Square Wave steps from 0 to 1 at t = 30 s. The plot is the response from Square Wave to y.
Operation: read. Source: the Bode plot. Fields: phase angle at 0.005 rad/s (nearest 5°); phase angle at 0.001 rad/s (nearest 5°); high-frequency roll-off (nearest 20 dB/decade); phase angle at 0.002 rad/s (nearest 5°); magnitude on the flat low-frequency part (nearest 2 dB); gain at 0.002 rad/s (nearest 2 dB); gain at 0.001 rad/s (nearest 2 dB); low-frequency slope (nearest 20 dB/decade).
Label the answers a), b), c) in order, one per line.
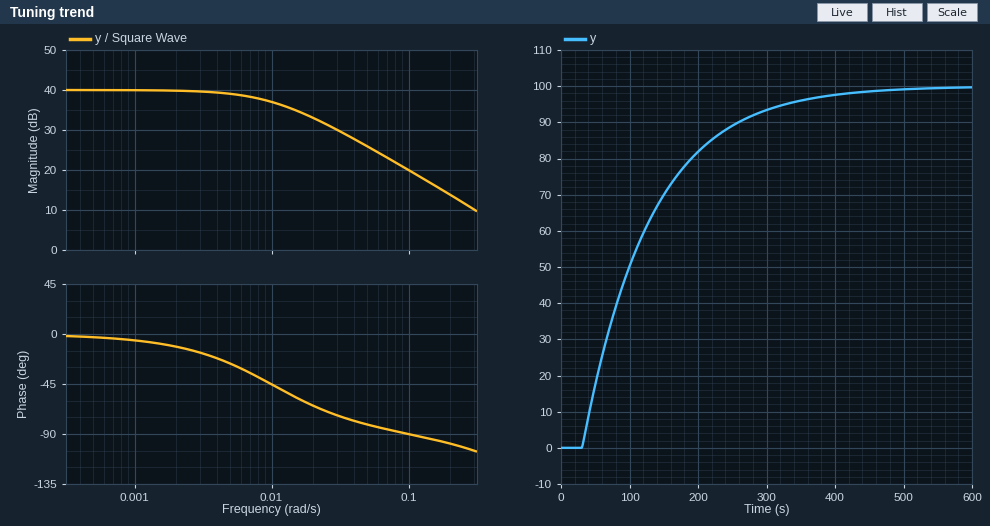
a) -25°
b) -5°
c) -20 dB/decade
d) -10°
e) 40 dB
f) 40 dB
g) 40 dB
h) 0 dB/decade
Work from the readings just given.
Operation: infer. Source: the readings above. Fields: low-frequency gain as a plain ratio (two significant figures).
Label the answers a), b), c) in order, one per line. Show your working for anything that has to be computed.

a) 10^(40 / 20) = 100
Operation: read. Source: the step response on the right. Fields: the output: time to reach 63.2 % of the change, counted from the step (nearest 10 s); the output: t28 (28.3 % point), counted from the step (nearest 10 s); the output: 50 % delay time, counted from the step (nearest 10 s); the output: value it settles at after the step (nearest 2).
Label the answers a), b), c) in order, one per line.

a) 100 s
b) 30 s
c) 70 s
d) 100
